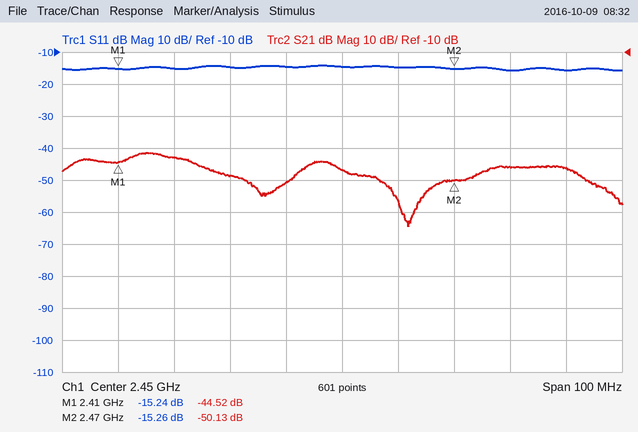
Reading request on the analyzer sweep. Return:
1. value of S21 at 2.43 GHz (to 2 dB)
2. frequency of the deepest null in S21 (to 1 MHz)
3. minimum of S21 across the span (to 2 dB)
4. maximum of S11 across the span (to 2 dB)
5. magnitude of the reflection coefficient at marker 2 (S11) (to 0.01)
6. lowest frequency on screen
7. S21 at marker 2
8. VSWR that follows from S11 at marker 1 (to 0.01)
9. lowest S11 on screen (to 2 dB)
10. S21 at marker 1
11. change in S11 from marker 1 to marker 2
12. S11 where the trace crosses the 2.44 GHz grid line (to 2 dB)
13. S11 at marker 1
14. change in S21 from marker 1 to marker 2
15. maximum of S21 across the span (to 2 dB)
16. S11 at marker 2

-48 dB
2.462 GHz
-64 dB
-14 dB
0.17
2.4 GHz
-50.13 dB
1.42
-16 dB
-44.52 dB
-0.02 dB
-14 dB
-15.24 dB
-5.61 dB
-42 dB
-15.26 dB
